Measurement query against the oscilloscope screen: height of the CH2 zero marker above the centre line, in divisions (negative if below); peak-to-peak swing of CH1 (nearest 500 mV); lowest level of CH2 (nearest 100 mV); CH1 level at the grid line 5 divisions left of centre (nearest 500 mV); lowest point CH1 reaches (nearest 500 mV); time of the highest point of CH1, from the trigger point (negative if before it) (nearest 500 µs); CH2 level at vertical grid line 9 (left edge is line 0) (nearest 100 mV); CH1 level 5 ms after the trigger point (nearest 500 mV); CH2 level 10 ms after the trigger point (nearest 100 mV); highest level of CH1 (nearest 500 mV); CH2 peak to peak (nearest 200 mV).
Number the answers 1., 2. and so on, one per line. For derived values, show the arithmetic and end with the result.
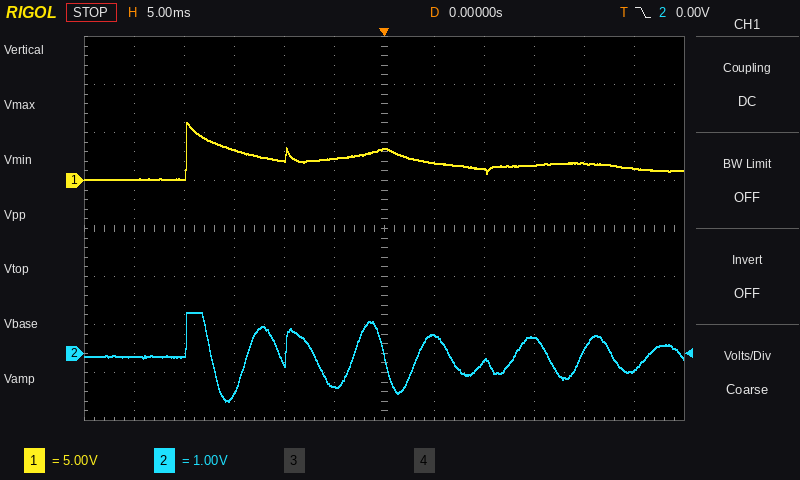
1. -2.6 div
2. 6.0 V − (0.0 V) = 6.0 V
3. -1.0 V
4. 0.0 V
5. 0.0 V
6. -19.5 ms
7. 300 mV
8. 2.0 V
9. -200 mV
10. 6.0 V
11. 1.8 V
